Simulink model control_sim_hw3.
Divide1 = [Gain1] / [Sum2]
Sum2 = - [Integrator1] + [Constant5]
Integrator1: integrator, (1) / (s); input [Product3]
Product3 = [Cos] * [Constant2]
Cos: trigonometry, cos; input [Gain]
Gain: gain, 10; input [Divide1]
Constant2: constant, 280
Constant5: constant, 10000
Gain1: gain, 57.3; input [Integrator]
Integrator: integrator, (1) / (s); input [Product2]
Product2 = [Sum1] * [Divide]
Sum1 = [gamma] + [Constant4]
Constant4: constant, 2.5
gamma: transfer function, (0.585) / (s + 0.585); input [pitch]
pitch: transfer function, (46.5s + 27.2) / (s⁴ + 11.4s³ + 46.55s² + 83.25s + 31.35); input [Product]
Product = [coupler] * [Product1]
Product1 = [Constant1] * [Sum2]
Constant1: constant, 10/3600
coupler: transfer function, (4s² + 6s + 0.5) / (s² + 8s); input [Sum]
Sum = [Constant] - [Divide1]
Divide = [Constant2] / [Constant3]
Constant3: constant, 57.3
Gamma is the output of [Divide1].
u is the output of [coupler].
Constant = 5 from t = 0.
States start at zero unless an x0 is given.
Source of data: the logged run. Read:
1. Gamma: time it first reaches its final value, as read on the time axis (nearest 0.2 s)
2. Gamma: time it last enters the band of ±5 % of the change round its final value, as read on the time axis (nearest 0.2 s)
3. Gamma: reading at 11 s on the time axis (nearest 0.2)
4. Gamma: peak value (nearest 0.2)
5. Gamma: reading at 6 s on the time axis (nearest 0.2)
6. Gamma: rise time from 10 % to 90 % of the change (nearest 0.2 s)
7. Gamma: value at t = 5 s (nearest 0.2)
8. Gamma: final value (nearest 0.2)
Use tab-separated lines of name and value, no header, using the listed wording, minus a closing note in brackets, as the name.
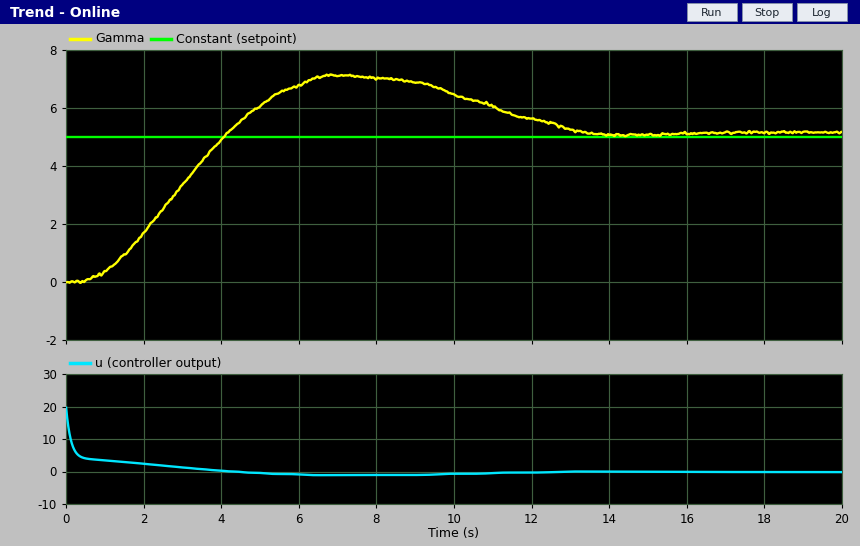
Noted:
Gamma: time it first reaches its final value, as read on the time axis	4.2 s
Gamma: time it last enters the band of ±5 % of the change round its final value, as read on the time axis	12.6 s
Gamma: reading at 11 s on the time axis	6.0
Gamma: peak value	7.2
Gamma: reading at 6 s on the time axis	6.8
Gamma: rise time from 10 % to 90 % of the change	2.6 s
Gamma: value at t = 5 s	6.0
Gamma: final value	5.2
